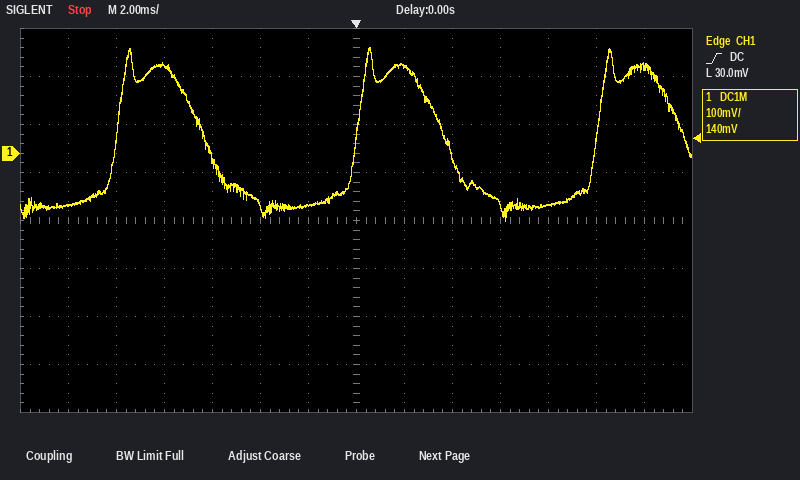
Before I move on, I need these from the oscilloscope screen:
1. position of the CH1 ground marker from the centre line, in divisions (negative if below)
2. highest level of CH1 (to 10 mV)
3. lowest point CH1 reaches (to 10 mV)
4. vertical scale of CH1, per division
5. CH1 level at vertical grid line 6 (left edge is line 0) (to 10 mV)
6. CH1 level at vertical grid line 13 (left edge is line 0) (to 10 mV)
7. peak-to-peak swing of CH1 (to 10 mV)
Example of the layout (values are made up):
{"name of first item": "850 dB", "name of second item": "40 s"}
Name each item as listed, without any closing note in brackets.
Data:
{"position of the CH1 ground marker from the centre line, in divisions": "+1.4 div", "highest level of CH1": "220 mV", "lowest point CH1 reaches": "-140 mV", "vertical scale of CH1, per division": "100 mV", "CH1 level at vertical grid line 6 (left edge is line 0)": "-110 mV", "CH1 level at vertical grid line 13 (left edge is line 0)": "180 mV", "peak-to-peak swing of CH1": "360 mV"}
